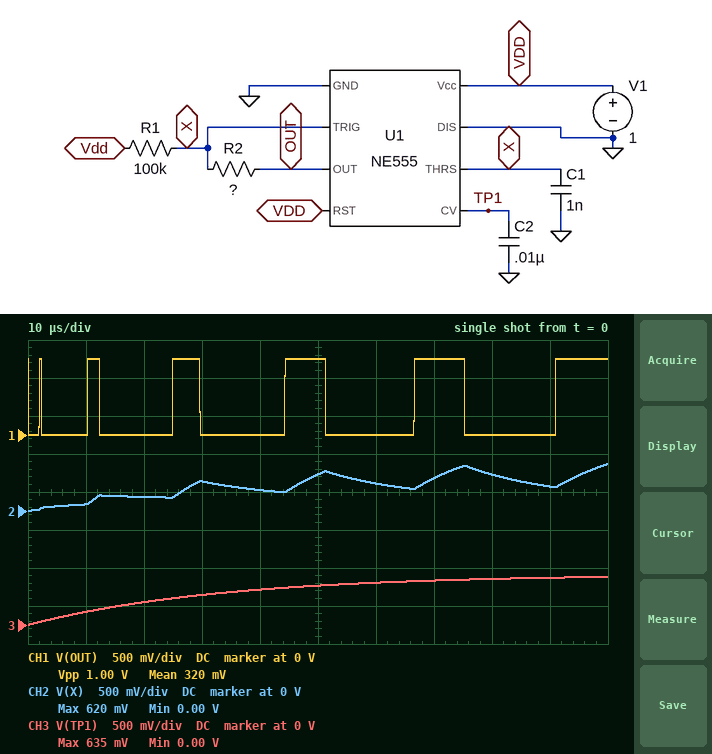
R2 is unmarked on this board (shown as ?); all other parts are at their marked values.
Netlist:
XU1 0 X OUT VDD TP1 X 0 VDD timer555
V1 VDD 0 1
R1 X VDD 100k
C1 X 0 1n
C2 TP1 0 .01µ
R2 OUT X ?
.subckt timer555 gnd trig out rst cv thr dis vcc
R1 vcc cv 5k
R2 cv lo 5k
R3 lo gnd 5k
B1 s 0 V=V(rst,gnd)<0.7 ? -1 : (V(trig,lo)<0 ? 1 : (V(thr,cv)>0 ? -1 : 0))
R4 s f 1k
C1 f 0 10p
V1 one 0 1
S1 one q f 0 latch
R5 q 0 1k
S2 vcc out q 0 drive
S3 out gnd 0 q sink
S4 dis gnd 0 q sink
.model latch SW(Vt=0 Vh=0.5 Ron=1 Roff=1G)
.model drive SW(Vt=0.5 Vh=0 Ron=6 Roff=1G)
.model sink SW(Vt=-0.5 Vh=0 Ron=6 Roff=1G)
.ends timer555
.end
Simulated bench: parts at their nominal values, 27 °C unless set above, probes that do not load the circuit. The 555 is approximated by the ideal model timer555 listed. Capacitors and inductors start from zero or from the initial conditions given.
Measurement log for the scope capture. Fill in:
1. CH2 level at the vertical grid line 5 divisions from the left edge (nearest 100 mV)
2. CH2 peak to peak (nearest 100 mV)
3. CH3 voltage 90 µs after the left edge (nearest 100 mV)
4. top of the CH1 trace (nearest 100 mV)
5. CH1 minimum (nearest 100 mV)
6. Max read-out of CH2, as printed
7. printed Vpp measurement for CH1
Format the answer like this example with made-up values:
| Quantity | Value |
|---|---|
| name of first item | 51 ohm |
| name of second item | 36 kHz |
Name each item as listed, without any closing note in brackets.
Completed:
| Quantity | Value |
|---|---|
| CH2 level at the vertical grid line 5 divisions from the left edge | 500 mV |
| CH2 peak to peak | 600 mV |
| CH3 voltage 90 µs after the left edge | 600 mV |
| top of the CH1 trace | 1.0 V |
| CH1 minimum | 0 V |
| Max read-out of CH2, as printed | 620 mV |
| printed Vpp measurement for CH1 | 1.00 V |
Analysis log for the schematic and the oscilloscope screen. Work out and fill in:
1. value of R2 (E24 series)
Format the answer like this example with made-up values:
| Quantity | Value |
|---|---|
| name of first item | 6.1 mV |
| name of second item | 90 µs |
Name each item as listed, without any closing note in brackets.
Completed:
| Quantity | Value |
|---|---|
| value of R2 | 18 kΩ |
